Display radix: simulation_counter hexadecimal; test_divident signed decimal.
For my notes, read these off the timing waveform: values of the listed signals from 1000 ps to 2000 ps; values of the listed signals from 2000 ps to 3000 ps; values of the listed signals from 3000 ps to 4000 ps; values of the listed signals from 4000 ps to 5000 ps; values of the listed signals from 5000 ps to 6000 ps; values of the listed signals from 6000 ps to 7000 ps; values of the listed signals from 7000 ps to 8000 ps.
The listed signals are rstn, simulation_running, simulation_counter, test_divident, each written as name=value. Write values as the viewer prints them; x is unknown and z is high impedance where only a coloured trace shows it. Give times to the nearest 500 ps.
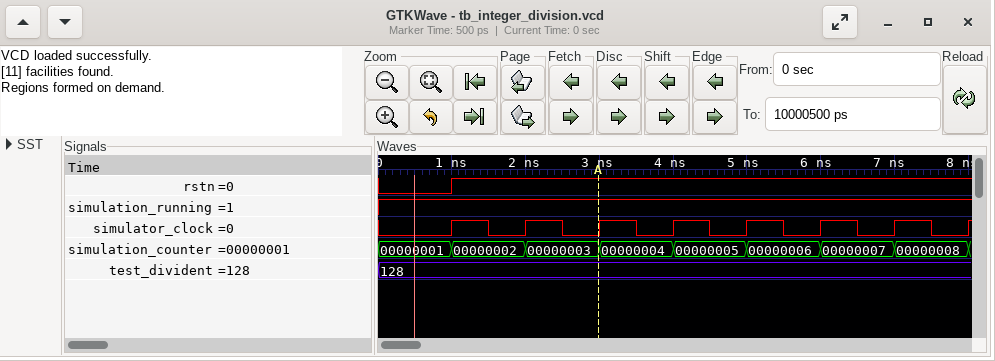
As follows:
rstn=1, simulation_running=1, simulation_counter=00000002, test_divident=128
rstn=1, simulation_running=1, simulation_counter=00000003, test_divident=128
rstn=1, simulation_running=1, simulation_counter=00000004, test_divident=128
rstn=1, simulation_running=1, simulation_counter=00000005, test_divident=128
rstn=1, simulation_running=1, simulation_counter=00000006, test_divident=128
rstn=1, simulation_running=1, simulation_counter=00000007, test_divident=128
rstn=1, simulation_running=1, simulation_counter=00000008, test_divident=128
